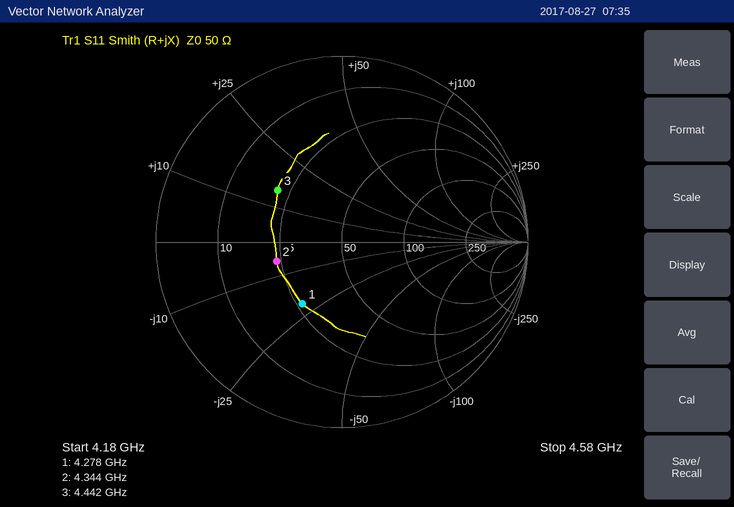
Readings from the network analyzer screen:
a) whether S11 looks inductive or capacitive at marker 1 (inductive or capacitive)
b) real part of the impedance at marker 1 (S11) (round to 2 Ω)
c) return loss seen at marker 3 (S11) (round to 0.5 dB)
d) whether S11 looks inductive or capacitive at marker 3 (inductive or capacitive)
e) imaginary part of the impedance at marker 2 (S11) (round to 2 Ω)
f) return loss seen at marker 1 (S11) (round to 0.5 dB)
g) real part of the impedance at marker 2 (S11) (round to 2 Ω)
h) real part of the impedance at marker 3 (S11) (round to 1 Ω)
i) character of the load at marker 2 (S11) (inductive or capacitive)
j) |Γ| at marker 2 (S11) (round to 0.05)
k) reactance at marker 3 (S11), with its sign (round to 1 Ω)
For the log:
capacitive
26 Ω
7.0 dB
inductive
-6 Ω
8.0 dB
24 Ω
21 Ω
capacitive
0.35
+15 Ω
